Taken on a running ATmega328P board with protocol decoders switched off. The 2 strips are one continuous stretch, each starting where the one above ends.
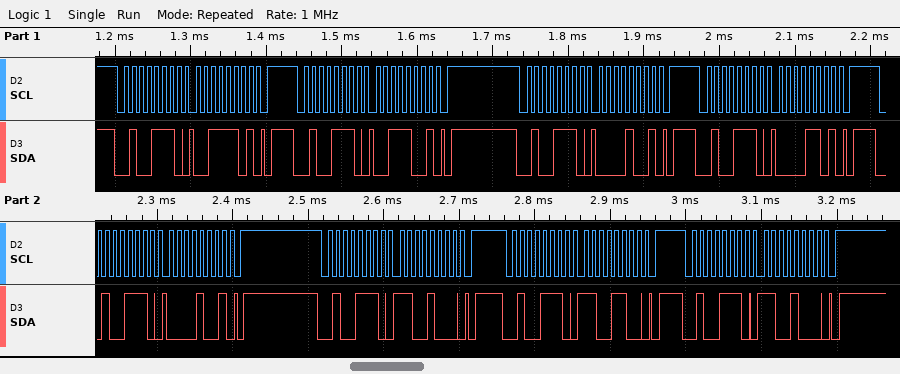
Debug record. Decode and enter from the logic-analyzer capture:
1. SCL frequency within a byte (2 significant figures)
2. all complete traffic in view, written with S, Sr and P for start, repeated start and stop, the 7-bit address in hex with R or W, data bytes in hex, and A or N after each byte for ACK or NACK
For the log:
100 kHz
S 27W A 3D A P S 27W A 39 A P S 27W A 09 A P S 27W A 0D A P S 27W A 09 A P S 27W A C8 A P S 27W A CC A P S 27W A C8 A P
